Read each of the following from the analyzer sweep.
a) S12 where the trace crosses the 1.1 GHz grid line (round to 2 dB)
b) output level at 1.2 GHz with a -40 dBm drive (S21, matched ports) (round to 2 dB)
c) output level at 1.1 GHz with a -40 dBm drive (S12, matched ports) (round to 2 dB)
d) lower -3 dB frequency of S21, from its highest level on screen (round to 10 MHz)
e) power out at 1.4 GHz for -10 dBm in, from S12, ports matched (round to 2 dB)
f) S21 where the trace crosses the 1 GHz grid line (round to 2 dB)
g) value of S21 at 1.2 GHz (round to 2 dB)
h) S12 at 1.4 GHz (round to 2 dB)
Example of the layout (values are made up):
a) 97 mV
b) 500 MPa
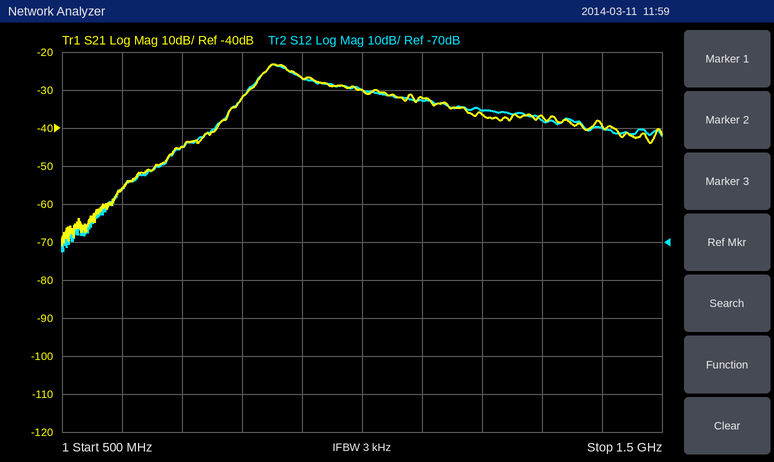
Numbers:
a) -32 dB
b) -76 dBm
c) -72 dBm
d) 830 MHz
e) -50 dBm
f) -30 dB
g) -36 dB
h) -40 dB
